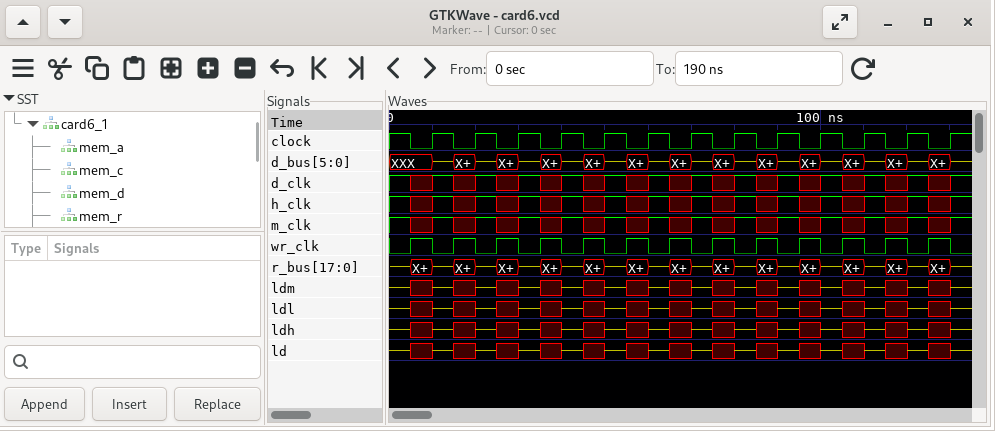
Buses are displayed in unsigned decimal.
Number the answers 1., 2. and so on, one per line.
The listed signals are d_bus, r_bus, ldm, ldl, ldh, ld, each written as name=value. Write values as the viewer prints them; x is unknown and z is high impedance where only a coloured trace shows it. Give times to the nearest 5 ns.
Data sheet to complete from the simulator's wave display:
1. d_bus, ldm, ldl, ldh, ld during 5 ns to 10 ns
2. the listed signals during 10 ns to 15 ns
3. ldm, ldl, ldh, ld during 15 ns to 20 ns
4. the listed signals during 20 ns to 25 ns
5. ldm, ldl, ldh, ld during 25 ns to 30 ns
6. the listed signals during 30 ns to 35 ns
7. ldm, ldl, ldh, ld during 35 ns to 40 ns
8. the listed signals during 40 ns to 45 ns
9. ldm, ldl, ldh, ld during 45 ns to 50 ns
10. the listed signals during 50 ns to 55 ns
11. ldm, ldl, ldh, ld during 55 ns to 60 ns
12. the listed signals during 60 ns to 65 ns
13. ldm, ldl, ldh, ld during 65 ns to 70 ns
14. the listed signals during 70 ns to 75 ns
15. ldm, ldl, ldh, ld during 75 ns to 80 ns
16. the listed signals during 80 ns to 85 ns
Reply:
1. d_bus=XXX, ldm=x, ldl=x, ldh=x, ld=x
2. d_bus=z, r_bus=z, ldm=z, ldl=z, ldh=z, ld=z
3. ldm=x, ldl=x, ldh=x, ld=x
4. d_bus=z, r_bus=z, ldm=z, ldl=z, ldh=z, ld=z
5. ldm=x, ldl=x, ldh=x, ld=x
6. d_bus=z, r_bus=z, ldm=z, ldl=z, ldh=z, ld=z
7. ldm=x, ldl=x, ldh=x, ld=x
8. d_bus=z, r_bus=z, ldm=z, ldl=z, ldh=z, ld=z
9. ldm=x, ldl=x, ldh=x, ld=x
10. d_bus=z, r_bus=z, ldm=z, ldl=z, ldh=z, ld=z
11. ldm=x, ldl=x, ldh=x, ld=x
12. d_bus=z, r_bus=z, ldm=z, ldl=z, ldh=z, ld=z
13. ldm=x, ldl=x, ldh=x, ld=x
14. d_bus=z, r_bus=z, ldm=z, ldl=z, ldh=z, ld=z
15. ldm=x, ldl=x, ldh=x, ld=x
16. d_bus=z, r_bus=z, ldm=z, ldl=z, ldh=z, ld=z
